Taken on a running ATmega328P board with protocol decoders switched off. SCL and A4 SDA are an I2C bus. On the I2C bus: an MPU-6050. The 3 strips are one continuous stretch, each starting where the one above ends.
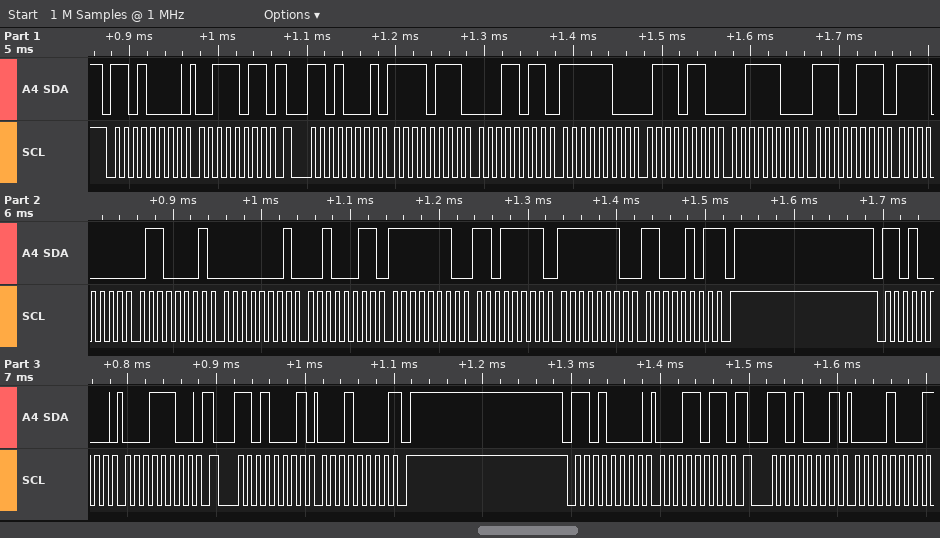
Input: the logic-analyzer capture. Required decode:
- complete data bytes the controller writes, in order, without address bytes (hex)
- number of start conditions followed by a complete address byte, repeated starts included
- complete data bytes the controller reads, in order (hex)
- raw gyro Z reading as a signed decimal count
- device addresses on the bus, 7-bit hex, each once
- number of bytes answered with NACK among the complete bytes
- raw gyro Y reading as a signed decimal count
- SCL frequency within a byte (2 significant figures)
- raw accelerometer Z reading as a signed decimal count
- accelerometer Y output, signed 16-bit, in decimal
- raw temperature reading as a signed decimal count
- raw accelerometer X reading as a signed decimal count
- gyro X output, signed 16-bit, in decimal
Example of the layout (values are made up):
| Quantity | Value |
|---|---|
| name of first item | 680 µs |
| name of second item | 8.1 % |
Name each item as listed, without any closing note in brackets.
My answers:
| Quantity | Value |
|---|---|
| complete data bytes the controller writes, in order, without address bytes | 3B 1C 1B |
| number of start conditions followed by a complete address byte, repeated starts included | 6 |
| complete data bytes the controller reads, in order | F7 1B FC 76 3C E7 F0 61 01 23 FE DF FE C5 10 08 |
| raw gyro Z reading as a signed decimal count | -315 |
| device addresses on the bus, 7-bit hex, each once | 0x68 |
| number of bytes answered with NACK among the complete bytes | 3 |
| raw gyro Y reading as a signed decimal count | -289 |
| SCL frequency within a byte | 100 kHz |
| raw accelerometer Z reading as a signed decimal count | 15591 |
| accelerometer Y output, signed 16-bit, in decimal | -906 |
| raw temperature reading as a signed decimal count | -3999 |
| raw accelerometer X reading as a signed decimal count | -2277 |
| gyro X output, signed 16-bit, in decimal | 291 |
